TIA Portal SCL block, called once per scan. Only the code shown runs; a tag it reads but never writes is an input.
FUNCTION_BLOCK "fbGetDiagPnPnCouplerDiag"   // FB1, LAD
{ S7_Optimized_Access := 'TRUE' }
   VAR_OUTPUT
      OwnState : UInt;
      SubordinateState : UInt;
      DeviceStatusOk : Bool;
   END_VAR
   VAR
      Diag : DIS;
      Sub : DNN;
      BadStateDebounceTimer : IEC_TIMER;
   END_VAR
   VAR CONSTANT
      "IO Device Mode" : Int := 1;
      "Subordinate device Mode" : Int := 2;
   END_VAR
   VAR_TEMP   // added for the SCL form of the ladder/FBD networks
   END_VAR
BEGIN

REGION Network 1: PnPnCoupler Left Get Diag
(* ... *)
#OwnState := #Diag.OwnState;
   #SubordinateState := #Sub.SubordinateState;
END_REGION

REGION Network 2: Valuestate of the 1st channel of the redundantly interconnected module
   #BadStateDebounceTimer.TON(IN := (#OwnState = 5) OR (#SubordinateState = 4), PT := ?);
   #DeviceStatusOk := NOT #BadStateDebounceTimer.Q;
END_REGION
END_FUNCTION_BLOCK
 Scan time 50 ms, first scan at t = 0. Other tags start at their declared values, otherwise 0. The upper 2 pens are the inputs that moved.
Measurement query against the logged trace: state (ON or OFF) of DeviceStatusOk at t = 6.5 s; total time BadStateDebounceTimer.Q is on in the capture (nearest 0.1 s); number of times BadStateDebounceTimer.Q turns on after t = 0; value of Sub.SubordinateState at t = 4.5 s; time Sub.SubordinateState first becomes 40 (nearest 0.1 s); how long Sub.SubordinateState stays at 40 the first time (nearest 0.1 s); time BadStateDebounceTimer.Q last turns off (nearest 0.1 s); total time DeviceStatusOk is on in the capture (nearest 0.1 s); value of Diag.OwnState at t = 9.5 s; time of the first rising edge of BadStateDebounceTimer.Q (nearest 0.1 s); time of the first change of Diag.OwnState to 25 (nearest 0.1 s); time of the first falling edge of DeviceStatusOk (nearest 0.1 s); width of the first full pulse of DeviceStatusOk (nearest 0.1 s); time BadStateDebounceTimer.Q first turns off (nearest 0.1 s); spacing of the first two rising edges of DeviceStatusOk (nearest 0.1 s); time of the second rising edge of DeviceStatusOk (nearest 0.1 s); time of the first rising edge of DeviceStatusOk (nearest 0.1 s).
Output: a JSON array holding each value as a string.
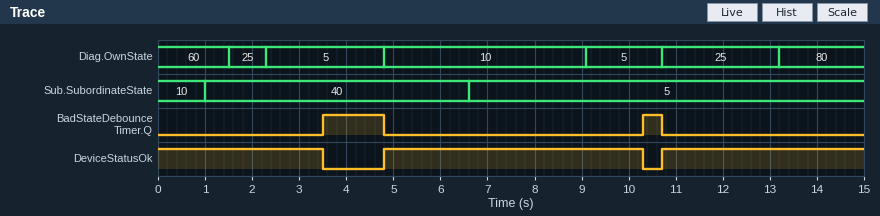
["ON", "1.7 s", "2", "40", "1.0 s", "5.6 s", "10.7 s", "13.3 s", "5", "3.5 s", "1.5 s", "3.5 s", "5.5 s", "4.8 s", "5.9 s", "10.7 s", "4.8 s"]
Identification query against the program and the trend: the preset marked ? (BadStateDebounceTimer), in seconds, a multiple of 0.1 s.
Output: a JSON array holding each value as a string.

["1.2 s"]
